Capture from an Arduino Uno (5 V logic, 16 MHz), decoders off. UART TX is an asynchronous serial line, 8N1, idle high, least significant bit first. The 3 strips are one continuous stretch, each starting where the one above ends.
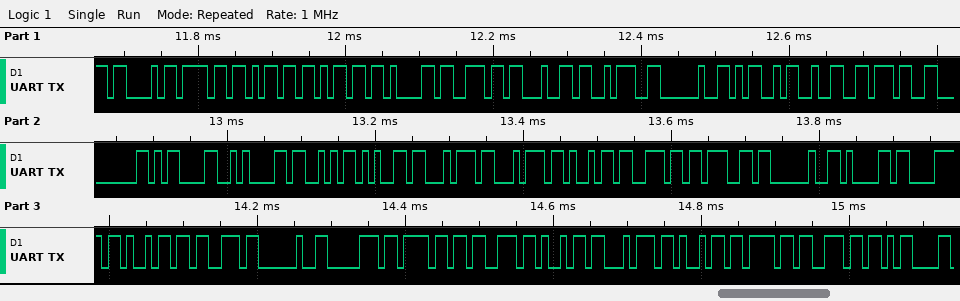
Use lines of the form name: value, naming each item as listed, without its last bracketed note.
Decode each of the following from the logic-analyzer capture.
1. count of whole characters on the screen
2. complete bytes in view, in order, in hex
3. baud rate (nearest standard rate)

count of whole characters on the screen: 37
complete bytes in view, in order, in hex: 43 6F 6D 6D 61 6E 64 3A 20 4D 32 37 00 0D 0A 53 65 74 74 69 6E 67 20 61 78 69 73 20 70 6F 73 69 74 69 6F 6E 0D
baud rate: 115200 baud
